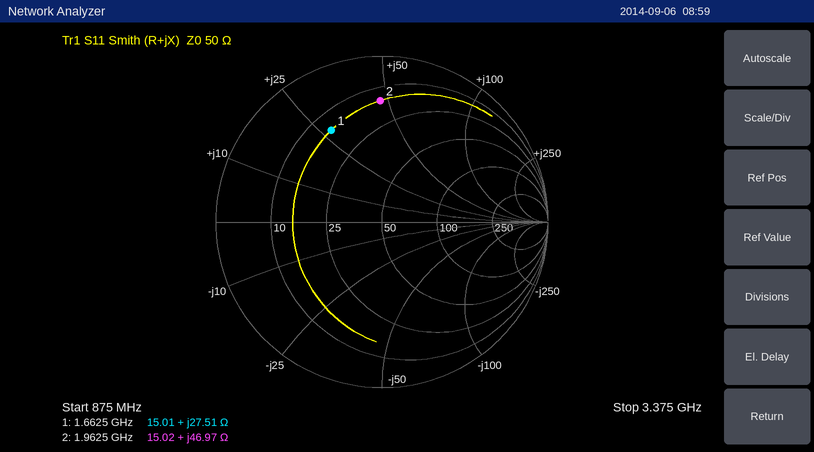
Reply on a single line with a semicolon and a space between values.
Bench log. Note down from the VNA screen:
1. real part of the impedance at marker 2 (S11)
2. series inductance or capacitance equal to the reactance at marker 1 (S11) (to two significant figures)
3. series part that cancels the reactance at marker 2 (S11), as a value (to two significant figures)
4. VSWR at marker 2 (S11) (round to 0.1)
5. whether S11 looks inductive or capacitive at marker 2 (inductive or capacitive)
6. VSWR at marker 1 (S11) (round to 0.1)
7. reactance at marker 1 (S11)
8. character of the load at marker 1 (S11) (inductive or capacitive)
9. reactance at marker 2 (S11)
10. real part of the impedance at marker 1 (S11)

15.02 Ω; 2.6 nH; 1.7 pF; 6.4; inductive; 4.4; +27.51 Ω; inductive; +46.97 Ω; 15.01 Ω
